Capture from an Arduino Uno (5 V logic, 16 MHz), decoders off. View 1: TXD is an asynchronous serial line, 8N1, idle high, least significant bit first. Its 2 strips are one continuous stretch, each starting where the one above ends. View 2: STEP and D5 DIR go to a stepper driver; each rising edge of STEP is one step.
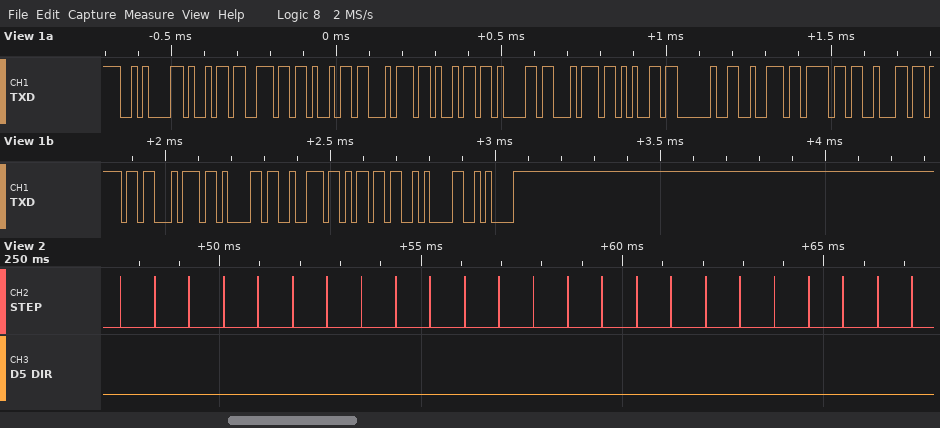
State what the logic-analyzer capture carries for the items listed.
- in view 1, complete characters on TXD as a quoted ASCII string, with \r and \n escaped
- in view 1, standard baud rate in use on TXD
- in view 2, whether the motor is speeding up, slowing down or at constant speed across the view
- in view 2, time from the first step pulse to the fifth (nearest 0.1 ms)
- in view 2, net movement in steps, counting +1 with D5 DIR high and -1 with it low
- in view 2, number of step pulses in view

"\ninitiate robotarm\n\n"
57600 baud
constant speed
3.4 ms
-24
24
